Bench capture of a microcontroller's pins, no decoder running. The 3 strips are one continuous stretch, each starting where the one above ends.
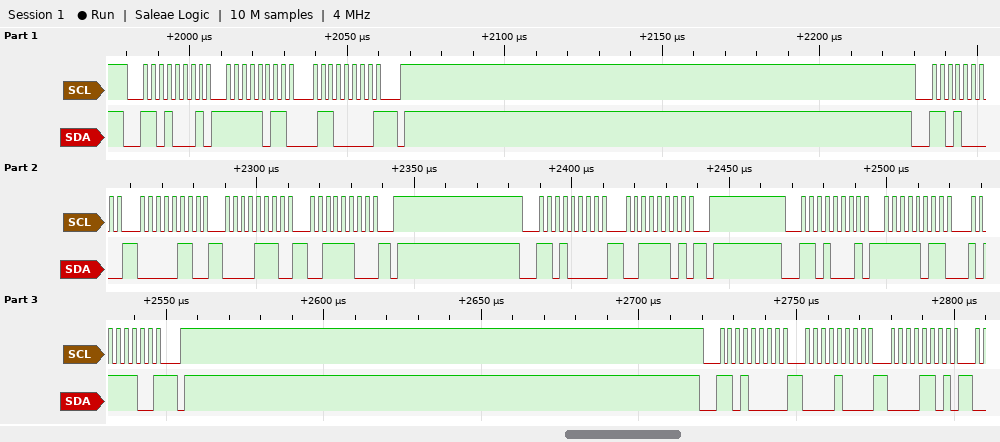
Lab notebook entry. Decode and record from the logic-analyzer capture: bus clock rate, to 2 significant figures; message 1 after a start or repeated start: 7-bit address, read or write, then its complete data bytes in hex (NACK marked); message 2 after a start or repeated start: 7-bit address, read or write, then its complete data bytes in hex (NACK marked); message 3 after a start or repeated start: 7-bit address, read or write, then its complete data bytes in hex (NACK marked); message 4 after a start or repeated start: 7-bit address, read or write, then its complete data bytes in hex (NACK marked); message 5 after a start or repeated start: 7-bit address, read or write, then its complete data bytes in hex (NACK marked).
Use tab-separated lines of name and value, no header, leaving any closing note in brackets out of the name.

bus clock rate, to 2 significant figures	400 kHz
message 1 after a start or repeated start: 7-bit address, read or write, then its complete data bytes in hex	0x68 read: FB 60 NACK
message 2 after a start or repeated start: 7-bit address, read or write, then its complete data bytes in hex	0x68 write: 06 0E 3C
message 3 after a start or repeated start: 7-bit address, read or write, then its complete data bytes in hex	0x68 write: 3D
message 4 after a start or repeated start: 7-bit address, read or write, then its complete data bytes in hex	0x68 read: FB BC NACK
message 5 after a start or repeated start: 7-bit address, read or write, then its complete data bytes in hex	0x68 write: 08 0D
